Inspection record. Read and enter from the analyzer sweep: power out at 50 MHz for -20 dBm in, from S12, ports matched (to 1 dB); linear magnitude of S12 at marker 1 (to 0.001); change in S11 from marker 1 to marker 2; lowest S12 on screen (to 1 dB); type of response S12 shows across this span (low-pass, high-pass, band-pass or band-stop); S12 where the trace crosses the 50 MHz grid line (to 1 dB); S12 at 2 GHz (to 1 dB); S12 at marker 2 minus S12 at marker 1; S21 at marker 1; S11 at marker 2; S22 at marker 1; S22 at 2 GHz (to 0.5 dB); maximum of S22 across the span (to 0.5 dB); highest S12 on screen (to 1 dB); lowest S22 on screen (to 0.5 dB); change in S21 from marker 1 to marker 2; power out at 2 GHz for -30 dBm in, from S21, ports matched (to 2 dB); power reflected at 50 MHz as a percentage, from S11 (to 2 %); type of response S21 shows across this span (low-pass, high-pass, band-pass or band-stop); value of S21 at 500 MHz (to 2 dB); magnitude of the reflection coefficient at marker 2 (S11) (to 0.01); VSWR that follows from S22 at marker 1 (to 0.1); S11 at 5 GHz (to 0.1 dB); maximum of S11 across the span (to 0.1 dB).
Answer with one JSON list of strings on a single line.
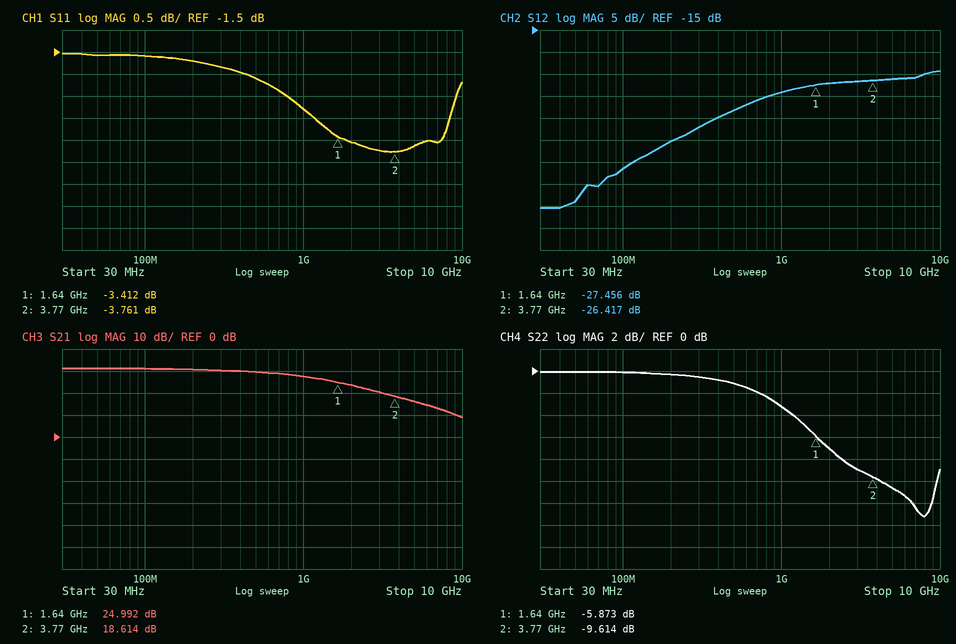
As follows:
["-74 dBm", "0.042", "-0.349 dB", "-55 dB", "high-pass", "-54 dB", "-27 dB", "1.039 dB", "24.992 dB", "-3.761 dB", "-5.873 dB", "-7.0 dB", "0.0 dB", "-24 dB", "-13.0 dB", "-6.378 dB", "-6 dBm", "70 %", "low-pass", "30 dB", "0.65", "3.1", "-3.6 dB", "-1.5 dB"]
